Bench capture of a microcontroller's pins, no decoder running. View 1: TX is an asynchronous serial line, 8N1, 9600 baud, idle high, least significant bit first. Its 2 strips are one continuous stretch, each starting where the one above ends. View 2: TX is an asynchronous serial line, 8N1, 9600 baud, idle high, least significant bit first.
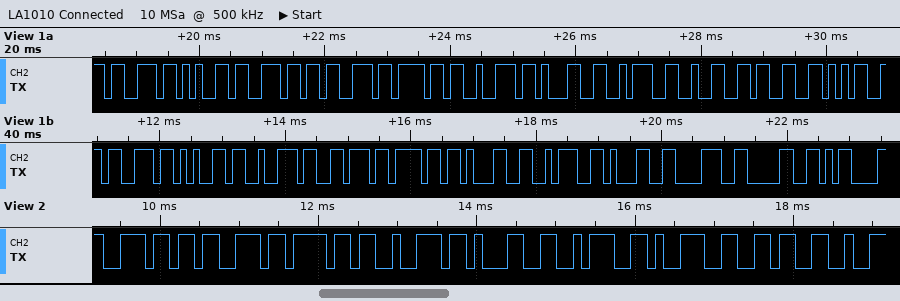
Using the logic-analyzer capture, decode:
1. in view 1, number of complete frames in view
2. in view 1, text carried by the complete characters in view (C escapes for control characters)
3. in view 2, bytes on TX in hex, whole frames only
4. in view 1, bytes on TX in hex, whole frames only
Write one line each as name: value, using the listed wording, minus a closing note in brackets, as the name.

in view 1, number of complete frames in view: 22
in view 1, text carried by the complete characters in view: "sensor1:235servo1:180\r"
in view 2, bytes on TX in hex, whole frames only: 6E 73 6F 72 31 3A 39 36
in view 1, bytes on TX in hex, whole frames only: 73 65 6E 73 6F 72 31 3A 32 33 35 73 65 72 76 6F 31 3A 31 38 30 0D
